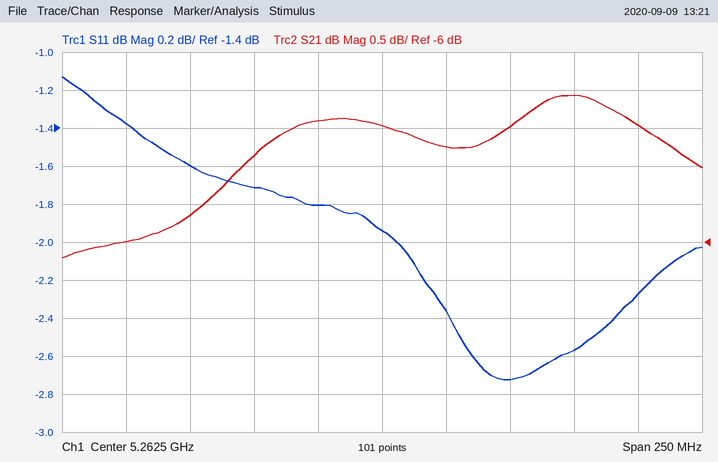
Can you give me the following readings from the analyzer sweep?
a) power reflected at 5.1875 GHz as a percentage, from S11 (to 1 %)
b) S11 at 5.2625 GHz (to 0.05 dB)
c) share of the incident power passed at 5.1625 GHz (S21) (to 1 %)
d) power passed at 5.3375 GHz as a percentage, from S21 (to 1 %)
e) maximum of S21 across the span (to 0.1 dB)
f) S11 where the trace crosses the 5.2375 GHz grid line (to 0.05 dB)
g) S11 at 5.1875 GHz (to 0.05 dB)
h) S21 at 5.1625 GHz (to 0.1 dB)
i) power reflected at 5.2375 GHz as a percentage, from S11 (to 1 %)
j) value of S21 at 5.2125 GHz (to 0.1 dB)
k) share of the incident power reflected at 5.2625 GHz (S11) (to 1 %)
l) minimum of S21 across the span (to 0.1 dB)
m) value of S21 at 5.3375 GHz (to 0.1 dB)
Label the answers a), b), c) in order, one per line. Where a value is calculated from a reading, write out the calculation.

a) 10^(-1.6/10) ≈ 69 %
b) -1.95 dB
c) 10^(-6/10) ≈ 25 %
d) 10^(-4.1/10) ≈ 39 %
e) -4.1 dB
f) -1.80 dB
g) -1.60 dB
h) -6.0 dB
i) 10^(-1.8/10) ≈ 66 %
j) -4.9 dB
k) 10^(-1.95/10) ≈ 64 %
l) -6.2 dB
m) -4.1 dB
